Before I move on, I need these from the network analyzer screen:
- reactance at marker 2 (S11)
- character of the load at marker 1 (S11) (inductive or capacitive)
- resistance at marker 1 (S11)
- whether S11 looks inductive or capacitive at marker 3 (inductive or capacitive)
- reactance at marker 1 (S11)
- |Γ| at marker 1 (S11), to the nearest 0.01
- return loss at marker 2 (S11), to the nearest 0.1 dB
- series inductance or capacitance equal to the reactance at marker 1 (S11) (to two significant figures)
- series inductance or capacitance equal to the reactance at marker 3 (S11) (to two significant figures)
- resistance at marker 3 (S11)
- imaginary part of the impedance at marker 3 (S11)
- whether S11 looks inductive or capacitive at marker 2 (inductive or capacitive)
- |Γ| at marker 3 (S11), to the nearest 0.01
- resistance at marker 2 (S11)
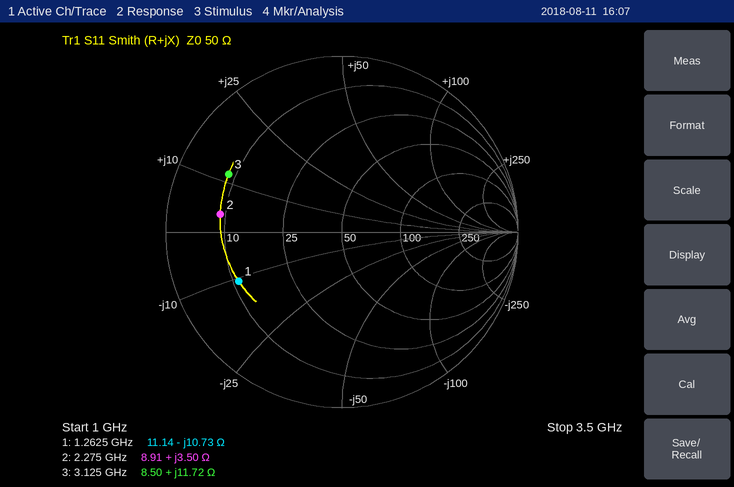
+3.50 Ω
capacitive
11.14 Ω
inductive
-10.73 Ω
0.65
3.1 dB
12 pF
600 pH
8.50 Ω
+11.72 Ω
inductive
0.72
8.91 Ω
